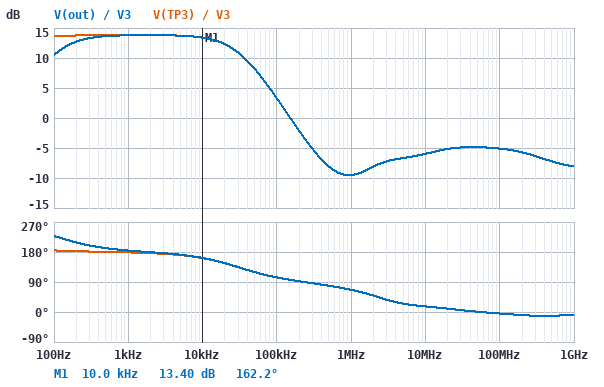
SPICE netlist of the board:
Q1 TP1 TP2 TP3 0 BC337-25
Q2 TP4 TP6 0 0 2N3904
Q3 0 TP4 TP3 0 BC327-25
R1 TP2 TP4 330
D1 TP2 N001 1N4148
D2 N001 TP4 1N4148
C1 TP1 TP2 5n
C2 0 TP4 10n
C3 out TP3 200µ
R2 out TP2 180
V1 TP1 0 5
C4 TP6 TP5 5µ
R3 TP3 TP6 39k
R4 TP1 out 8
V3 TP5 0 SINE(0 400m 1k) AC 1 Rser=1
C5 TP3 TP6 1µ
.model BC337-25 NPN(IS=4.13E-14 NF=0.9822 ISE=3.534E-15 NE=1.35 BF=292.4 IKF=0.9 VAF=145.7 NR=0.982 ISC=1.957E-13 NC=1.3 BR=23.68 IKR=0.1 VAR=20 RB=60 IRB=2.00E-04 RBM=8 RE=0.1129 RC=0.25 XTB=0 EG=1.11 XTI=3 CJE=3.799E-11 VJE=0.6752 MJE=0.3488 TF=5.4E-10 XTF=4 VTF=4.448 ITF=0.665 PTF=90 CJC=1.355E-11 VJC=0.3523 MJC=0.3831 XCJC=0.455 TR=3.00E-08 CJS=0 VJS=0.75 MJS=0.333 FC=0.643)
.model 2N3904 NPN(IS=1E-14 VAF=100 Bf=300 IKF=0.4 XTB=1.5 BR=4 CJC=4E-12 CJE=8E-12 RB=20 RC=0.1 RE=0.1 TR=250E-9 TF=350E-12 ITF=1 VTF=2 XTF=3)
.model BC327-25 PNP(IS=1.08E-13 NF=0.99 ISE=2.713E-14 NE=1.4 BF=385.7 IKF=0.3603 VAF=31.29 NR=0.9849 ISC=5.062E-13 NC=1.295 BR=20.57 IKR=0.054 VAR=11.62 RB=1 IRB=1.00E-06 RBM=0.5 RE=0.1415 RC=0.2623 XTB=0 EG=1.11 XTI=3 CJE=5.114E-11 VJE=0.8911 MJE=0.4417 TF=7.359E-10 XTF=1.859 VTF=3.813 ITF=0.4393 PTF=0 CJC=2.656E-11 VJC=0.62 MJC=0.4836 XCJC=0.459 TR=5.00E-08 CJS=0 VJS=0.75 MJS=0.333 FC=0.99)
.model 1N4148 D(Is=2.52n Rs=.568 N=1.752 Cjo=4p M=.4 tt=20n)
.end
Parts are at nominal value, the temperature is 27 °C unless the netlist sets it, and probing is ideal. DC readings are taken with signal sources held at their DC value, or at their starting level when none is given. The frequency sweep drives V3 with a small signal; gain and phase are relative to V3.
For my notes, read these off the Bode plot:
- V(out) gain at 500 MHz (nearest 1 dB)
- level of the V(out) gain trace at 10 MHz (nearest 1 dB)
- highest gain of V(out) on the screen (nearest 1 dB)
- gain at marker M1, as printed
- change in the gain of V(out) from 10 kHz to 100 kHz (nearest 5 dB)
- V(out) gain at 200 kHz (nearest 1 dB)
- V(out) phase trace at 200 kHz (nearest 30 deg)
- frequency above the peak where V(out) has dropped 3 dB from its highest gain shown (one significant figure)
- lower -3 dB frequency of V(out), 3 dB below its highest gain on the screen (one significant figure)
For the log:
-7 dB
-6 dB
14 dB
13.40 dB
-10 dB
-2 dB
90 deg
30 kHz
100 Hz
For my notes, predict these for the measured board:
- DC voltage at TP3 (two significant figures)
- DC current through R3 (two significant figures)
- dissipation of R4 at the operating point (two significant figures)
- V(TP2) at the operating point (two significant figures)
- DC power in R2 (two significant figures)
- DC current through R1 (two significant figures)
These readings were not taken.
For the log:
2.2 V
38 µA
1.0 mW
2.9 V
23 mW
4.1 mA
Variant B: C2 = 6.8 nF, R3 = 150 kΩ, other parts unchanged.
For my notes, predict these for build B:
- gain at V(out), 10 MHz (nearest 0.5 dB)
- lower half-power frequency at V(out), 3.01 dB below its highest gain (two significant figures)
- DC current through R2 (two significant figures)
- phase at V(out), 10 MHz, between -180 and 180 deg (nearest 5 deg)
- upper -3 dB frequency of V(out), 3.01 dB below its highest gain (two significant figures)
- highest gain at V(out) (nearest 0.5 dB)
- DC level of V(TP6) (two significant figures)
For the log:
-2.0 dB
97 Hz
5.4 mA
0 deg
30 kHz
12.5 dB
700 mV
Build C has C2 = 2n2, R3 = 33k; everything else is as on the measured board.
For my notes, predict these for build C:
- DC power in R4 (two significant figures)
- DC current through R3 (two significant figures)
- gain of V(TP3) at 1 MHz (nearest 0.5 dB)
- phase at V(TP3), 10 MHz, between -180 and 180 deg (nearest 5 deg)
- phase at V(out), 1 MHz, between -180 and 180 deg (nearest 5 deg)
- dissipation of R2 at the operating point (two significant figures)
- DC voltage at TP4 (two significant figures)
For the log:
1.1 mW
41 µA
-12.5 dB
35 deg
75 deg
26 mW
1.4 V
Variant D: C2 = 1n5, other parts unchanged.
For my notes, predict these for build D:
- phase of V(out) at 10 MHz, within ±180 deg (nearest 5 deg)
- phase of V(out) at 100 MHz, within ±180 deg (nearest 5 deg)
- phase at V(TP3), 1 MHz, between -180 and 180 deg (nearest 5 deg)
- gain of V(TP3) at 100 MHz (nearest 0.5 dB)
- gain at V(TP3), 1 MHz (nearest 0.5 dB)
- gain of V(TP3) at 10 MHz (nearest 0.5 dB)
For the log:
40 deg
0 deg
75 deg
-4.5 dB
-12.5 dB
-7.0 dB
